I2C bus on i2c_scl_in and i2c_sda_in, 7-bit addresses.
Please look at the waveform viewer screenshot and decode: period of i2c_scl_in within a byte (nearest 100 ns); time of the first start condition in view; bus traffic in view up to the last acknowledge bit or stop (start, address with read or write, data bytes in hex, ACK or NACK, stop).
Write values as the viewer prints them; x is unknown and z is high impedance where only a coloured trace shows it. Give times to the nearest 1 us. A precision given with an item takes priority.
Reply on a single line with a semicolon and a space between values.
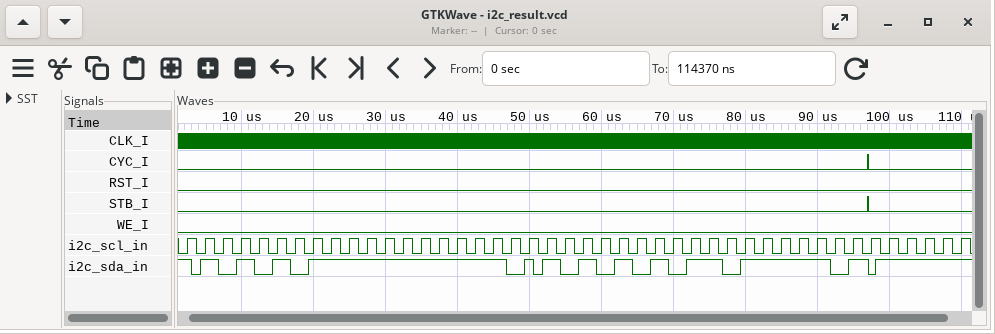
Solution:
2500 ns; 3 us; start, address 55 read NACK, FF ACK, repeated start, address 55 write NACK, BE NACK, stop
